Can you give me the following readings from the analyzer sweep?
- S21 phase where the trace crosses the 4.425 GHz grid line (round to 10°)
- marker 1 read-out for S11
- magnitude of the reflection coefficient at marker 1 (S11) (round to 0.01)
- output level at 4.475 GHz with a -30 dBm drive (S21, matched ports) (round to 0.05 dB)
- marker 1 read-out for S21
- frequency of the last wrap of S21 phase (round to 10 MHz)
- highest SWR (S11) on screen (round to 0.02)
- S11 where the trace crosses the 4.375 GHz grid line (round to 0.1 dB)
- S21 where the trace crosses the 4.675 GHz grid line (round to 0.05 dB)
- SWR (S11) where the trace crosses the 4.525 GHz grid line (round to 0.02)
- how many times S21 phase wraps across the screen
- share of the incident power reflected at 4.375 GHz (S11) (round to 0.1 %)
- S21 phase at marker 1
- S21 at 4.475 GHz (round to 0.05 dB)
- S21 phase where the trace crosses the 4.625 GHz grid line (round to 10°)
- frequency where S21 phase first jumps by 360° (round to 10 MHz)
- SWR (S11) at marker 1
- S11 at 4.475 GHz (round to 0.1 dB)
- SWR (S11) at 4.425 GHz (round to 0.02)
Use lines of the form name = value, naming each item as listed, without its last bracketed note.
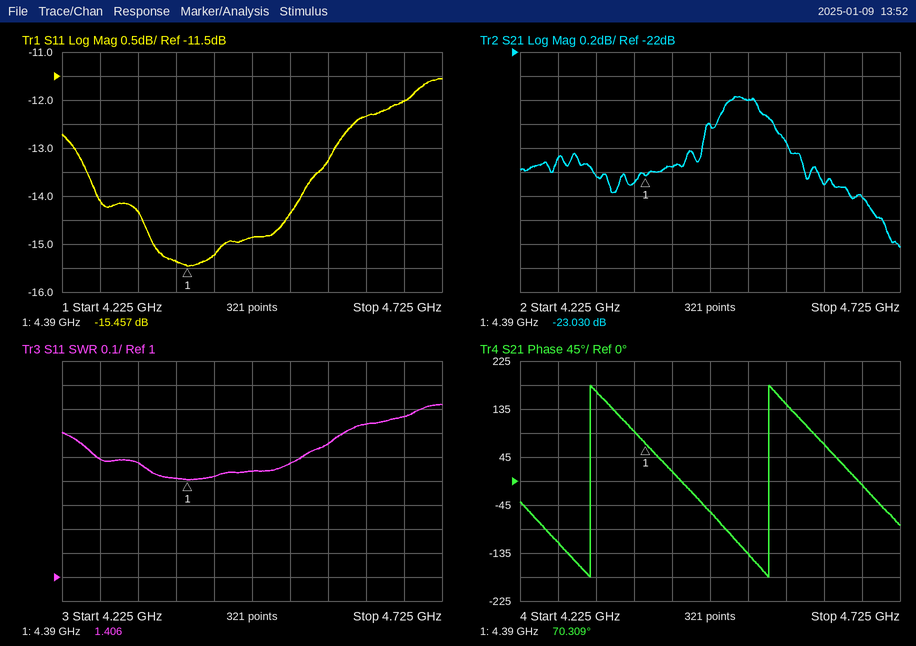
S21 phase where the trace crosses the 4.425 GHz grid line = 20°
marker 1 read-out for S11 = -15.457 dB
magnitude of the reflection coefficient at marker 1 (S11) = 0.17
output level at 4.475 GHz with a -30 dBm drive (S21, matched ports) = -52.60 dBm
marker 1 read-out for S21 = -23.030 dB
frequency of the last wrap of S21 phase = 4.55 GHz
highest SWR (S11) on screen = 1.72
S11 where the trace crosses the 4.375 GHz grid line = -15.4 dB
S21 where the trace crosses the 4.675 GHz grid line = -23.20 dB
SWR (S11) where the trace crosses the 4.525 GHz grid line = 1.48
how many times S21 phase wraps across the screen = 2
share of the incident power reflected at 4.375 GHz (S11) = 2.9 %
S21 phase at marker 1 = 70.309°
S21 at 4.475 GHz = -22.60 dB
S21 phase where the trace crosses the 4.625 GHz grid line = 70°
frequency where S21 phase first jumps by 360° = 4.32 GHz
SWR (S11) at marker 1 = 1.406
S11 at 4.475 GHz = -14.9 dB
SWR (S11) at 4.425 GHz = 1.42
